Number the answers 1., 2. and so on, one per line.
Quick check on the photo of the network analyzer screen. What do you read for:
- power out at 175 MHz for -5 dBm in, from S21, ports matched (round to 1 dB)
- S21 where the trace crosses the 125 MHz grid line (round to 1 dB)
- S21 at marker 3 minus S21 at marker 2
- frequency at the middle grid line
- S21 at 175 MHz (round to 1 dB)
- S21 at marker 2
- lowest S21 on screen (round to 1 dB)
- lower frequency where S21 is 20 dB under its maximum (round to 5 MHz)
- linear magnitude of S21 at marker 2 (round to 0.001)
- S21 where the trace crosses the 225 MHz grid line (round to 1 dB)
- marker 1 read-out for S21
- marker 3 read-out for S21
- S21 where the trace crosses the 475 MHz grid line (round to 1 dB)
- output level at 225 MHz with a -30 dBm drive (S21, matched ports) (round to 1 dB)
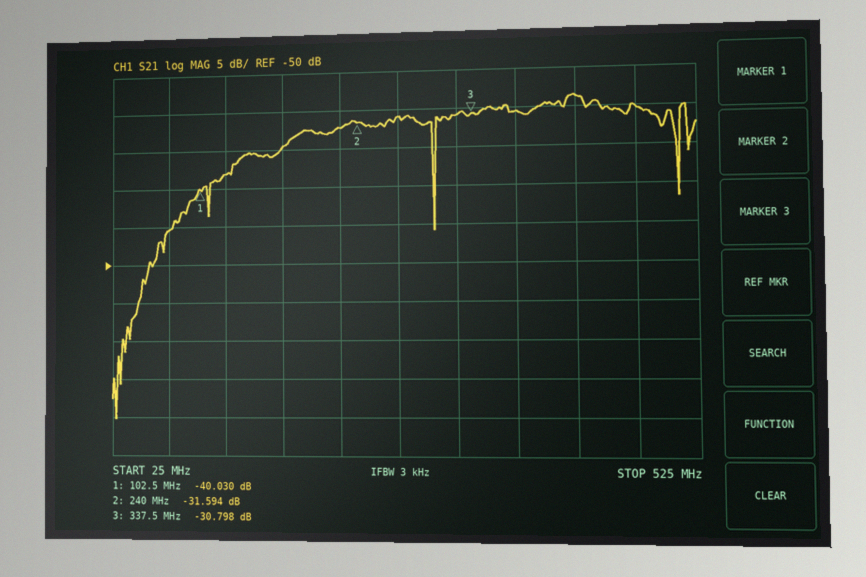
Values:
1. -40 dBm
2. -38 dB
3. 0.796 dB
4. 275 MHz
5. -35 dB
6. -31.594 dB
7. -70 dB
8. 65 MHz
9. 0.026
10. -32 dB
11. -40.030 dB
12. -30.798 dB
13. -30 dB
14. -62 dBm
